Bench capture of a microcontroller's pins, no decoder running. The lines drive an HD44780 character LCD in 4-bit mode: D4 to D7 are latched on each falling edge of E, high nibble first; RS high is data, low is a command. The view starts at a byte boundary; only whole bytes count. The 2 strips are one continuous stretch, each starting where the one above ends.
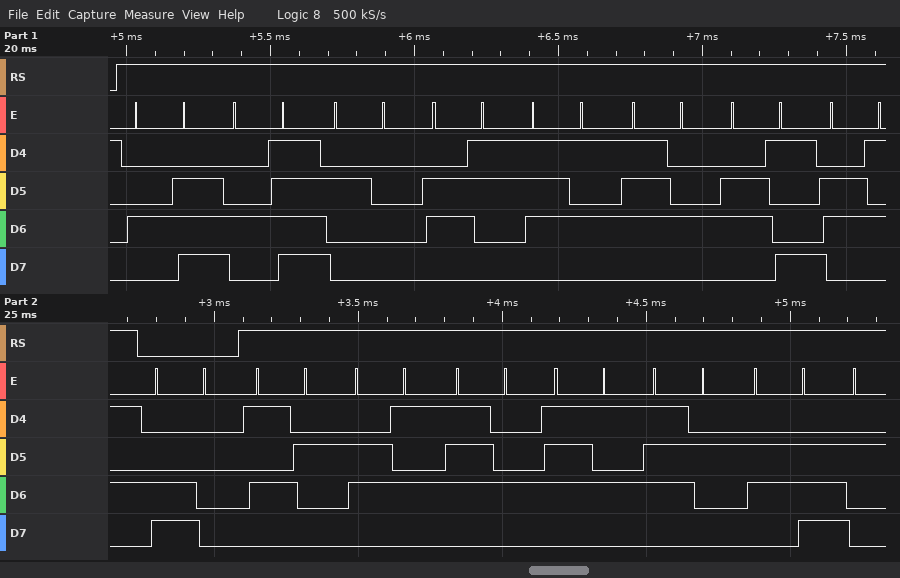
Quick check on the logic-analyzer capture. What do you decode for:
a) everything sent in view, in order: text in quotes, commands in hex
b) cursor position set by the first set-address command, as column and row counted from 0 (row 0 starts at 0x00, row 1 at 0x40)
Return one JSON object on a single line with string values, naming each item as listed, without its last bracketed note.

{"everything sent in view, in order: text in quotes, commands in hex": "\"NO cutie\" 0xC0 \"Return\"", "cursor position set by the first set-address command, as column and row counted from 0": "column 0, row 1"}
